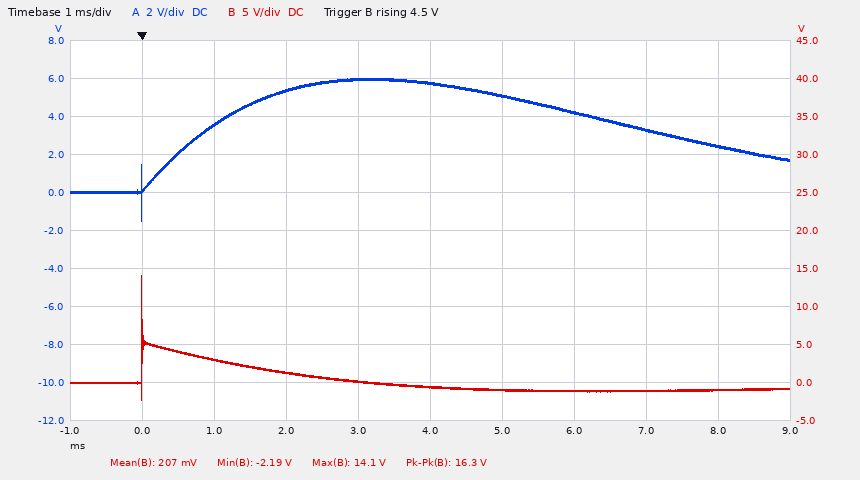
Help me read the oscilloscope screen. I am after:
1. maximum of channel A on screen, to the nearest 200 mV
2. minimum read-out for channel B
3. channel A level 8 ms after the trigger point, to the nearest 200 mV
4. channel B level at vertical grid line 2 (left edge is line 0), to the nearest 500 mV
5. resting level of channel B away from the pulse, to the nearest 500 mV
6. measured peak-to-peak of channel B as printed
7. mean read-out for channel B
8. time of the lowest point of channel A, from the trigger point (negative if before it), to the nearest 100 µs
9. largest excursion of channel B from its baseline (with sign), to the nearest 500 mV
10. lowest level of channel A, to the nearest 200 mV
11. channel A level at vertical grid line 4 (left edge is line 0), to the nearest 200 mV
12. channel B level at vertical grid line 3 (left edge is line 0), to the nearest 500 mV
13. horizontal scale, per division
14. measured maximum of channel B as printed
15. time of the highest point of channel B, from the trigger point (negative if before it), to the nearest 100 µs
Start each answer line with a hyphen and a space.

- 6.0 V
- -2.19 V
- 2.4 V
- 3.0 V
- -1.0 V
- 16.3 V
- 207 mV
- 0.0 ms
- +15.0 V
- -1.4 V
- 6.0 V
- 1.5 V
- 1 ms
- 14.1 V
- 0.0 ms
